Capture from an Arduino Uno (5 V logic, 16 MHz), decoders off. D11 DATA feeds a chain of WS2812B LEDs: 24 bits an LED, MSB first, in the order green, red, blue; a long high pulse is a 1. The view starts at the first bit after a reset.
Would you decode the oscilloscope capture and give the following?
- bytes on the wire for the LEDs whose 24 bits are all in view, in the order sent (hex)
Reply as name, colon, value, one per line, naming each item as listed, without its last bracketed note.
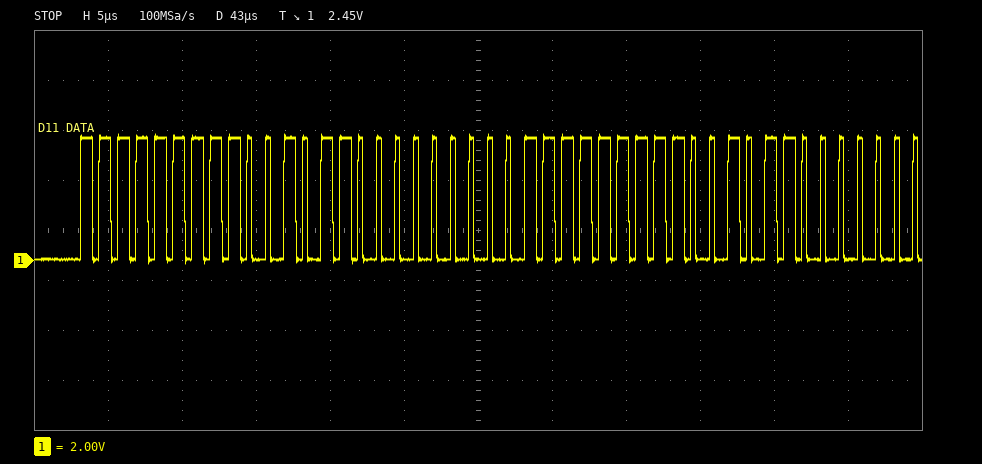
bytes on the wire for the LEDs whose 24 bits are all in view, in the order sent: FF 96 00
